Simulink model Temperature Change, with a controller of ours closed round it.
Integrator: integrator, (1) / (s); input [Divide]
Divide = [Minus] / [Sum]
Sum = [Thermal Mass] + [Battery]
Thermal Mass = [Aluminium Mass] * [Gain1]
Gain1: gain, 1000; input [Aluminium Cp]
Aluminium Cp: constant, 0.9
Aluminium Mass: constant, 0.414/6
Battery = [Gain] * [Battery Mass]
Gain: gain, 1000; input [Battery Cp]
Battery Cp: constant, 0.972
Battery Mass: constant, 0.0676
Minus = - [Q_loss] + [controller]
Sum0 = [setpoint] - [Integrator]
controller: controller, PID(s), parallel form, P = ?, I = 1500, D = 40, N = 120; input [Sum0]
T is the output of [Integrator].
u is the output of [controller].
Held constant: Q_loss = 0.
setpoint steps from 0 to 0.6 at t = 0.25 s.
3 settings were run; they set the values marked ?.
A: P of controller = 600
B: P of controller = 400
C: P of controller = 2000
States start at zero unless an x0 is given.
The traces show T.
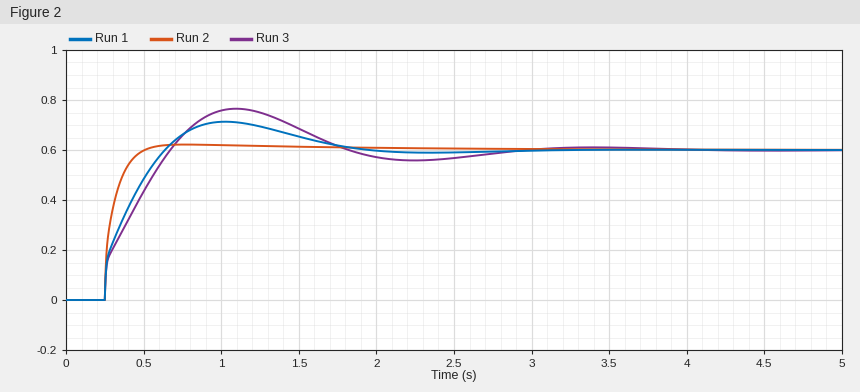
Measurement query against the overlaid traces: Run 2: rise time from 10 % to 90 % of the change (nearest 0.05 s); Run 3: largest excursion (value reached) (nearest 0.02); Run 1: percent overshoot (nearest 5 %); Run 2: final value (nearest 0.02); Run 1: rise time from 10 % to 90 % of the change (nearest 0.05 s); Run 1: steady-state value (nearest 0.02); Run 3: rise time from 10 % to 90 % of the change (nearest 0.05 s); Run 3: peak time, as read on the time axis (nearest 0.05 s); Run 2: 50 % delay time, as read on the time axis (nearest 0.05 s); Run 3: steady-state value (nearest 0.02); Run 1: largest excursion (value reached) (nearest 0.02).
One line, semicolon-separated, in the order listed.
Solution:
0.15 s; 0.76; 20 %; 0.60; 0.30 s; 0.60; 0.35 s; 1.10 s; 0.30 s; 0.60; 0.72
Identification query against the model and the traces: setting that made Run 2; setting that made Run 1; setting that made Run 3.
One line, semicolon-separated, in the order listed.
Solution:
C; A; B
